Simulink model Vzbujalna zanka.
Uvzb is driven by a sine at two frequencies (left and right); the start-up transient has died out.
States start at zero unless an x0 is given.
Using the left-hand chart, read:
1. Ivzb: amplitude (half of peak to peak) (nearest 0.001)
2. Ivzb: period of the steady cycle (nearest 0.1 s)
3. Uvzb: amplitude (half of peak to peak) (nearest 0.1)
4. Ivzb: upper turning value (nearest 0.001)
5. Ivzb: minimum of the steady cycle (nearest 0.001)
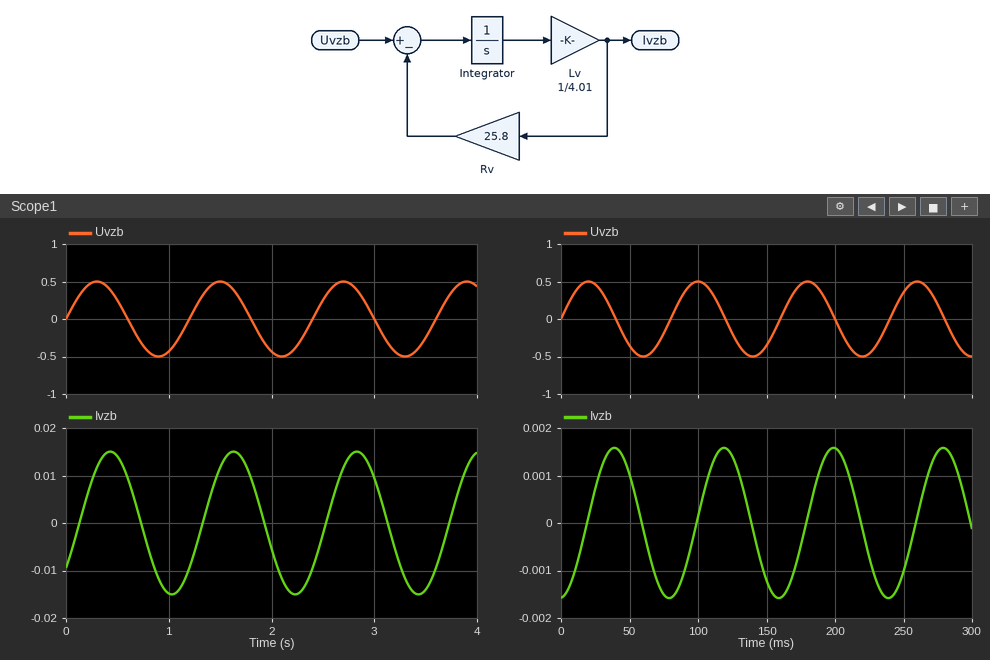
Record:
0.015
1.2 s
0.5
0.015
-0.015
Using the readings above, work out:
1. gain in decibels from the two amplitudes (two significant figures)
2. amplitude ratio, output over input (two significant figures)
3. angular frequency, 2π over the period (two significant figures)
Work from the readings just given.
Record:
-30 dB
0.030
5.2 rad/s
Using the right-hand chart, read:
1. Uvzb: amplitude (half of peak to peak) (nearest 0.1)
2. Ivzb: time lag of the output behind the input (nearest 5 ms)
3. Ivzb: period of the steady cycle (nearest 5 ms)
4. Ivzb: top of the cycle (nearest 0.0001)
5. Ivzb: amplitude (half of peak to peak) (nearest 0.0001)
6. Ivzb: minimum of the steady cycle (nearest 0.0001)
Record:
0.5
20 ms
80 ms
0.0016
0.0016
-0.0016
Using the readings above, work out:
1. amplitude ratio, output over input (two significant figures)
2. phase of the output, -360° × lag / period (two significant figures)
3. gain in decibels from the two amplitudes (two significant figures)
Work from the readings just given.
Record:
0.0032
-90°
-50 dB
